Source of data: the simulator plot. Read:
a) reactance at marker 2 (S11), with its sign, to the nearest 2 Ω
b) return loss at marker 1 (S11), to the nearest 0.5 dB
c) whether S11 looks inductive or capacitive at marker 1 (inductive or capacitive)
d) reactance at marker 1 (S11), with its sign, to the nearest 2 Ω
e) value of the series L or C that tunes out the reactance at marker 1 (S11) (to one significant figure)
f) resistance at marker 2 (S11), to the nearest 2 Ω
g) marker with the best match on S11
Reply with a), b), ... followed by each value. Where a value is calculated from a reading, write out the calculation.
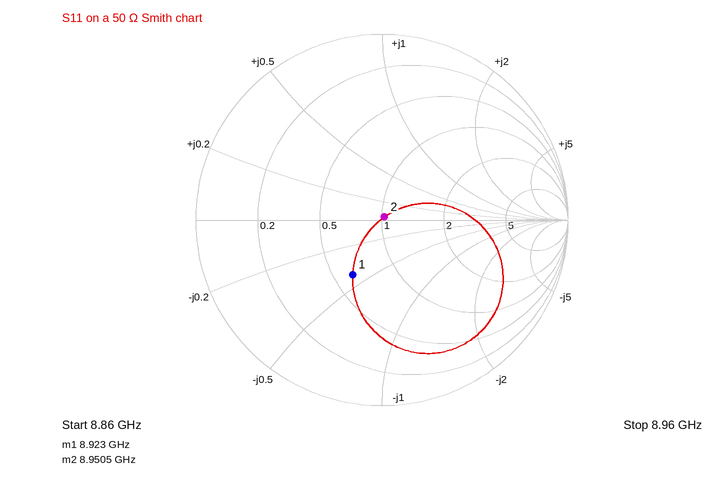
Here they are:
a) +2 Ω
b) 9.5 dB
c) capacitive
d) -20 Ω
e) L = 20 Ω/(2π × 8.923 GHz) ≈ 357 pH, so 400 pH to one significant figure
f) 52 Ω
g) marker 2
